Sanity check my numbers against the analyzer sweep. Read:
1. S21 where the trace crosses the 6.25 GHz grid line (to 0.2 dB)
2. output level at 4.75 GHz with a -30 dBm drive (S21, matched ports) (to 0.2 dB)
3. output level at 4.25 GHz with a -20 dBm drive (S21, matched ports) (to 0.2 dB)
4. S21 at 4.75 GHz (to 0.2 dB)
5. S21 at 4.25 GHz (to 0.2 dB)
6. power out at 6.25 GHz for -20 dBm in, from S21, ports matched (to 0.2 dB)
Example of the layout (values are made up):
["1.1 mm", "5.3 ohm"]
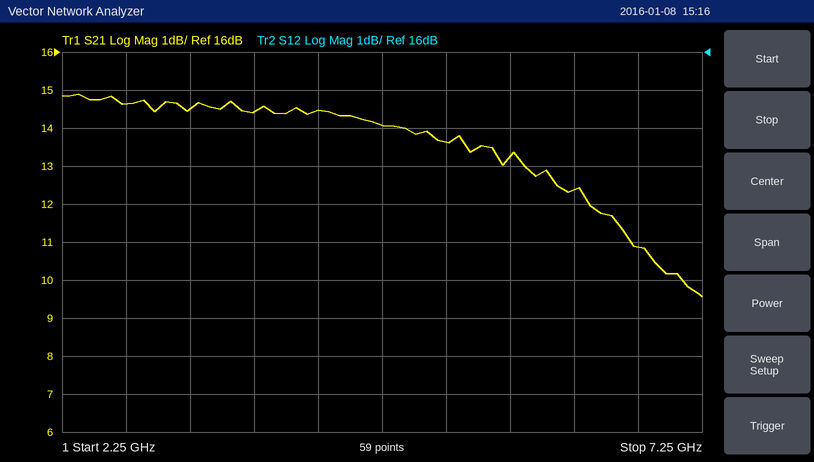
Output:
["12.4 dB", "-16.0 dBm", "-5.6 dBm", "14.0 dB", "14.4 dB", "-7.6 dBm"]
